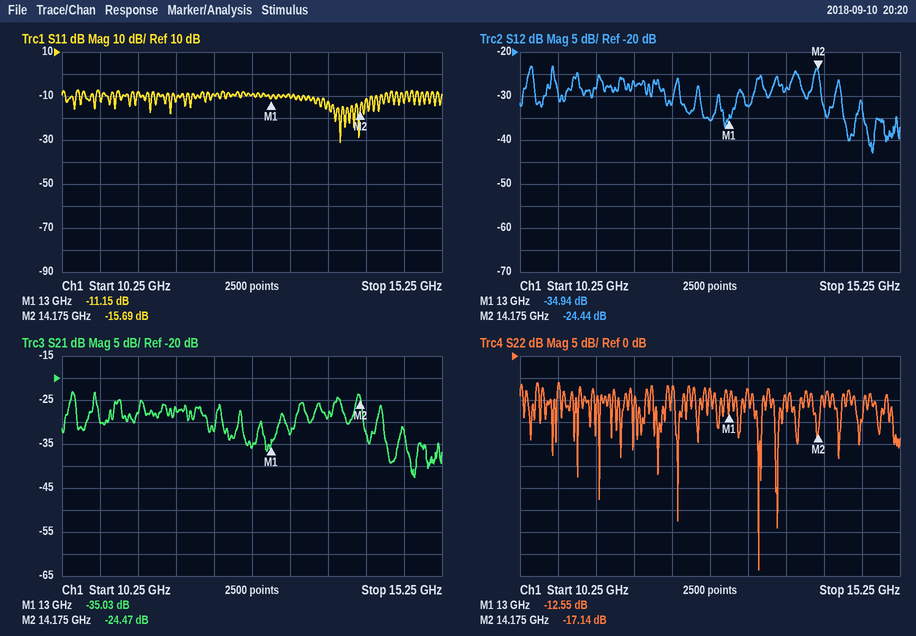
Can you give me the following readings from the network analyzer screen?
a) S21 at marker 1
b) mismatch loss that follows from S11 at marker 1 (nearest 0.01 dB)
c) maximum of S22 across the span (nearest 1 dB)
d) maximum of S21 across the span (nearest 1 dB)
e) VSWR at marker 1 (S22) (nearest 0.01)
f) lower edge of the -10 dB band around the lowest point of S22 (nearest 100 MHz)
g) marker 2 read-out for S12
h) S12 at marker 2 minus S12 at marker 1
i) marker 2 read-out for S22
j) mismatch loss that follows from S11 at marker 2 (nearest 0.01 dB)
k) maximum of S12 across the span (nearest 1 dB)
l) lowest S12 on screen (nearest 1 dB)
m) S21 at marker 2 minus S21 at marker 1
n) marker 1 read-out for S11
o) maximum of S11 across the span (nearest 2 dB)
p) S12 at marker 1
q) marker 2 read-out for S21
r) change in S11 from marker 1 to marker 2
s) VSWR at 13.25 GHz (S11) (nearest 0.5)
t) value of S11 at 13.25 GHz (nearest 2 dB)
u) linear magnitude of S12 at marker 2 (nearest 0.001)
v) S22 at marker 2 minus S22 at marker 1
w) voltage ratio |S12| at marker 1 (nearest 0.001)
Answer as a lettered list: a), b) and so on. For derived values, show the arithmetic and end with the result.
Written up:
a) -35.03 dB
b) −10 log10(1 − 10^(-11.15/10)) ≈ 0.35 dB
c) -6 dB
d) -23 dB
e) (1 + 0.2358)/(1 − 0.2358) ≈ 1.62
f) 13.3 GHz
g) -24.44 dB
h) -24.44 − (-34.94) = 10.50 dB
i) -17.14 dB
j) −10 log10(1 − 10^(-15.69/10)) ≈ 0.12 dB
k) -23 dB
l) -43 dB
m) -24.47 − (-35.03) = 10.56 dB
n) -11.15 dB
o) -8 dB
p) -34.94 dB
q) -24.47 dB
r) -15.69 − (-11.15) = -4.54 dB
s) |Γ| = 10^(-10/20) = 0.3162; VSWR = (1 + 0.3162)/(1 − 0.3162) ≈ 1.92, so 2.0 to the nearest 0.5
t) -10 dB
u) 10^(-24.44/20) ≈ 0.060
v) -17.14 − (-12.55) = -4.59 dB
w) 10^(-34.94/20) ≈ 0.018
